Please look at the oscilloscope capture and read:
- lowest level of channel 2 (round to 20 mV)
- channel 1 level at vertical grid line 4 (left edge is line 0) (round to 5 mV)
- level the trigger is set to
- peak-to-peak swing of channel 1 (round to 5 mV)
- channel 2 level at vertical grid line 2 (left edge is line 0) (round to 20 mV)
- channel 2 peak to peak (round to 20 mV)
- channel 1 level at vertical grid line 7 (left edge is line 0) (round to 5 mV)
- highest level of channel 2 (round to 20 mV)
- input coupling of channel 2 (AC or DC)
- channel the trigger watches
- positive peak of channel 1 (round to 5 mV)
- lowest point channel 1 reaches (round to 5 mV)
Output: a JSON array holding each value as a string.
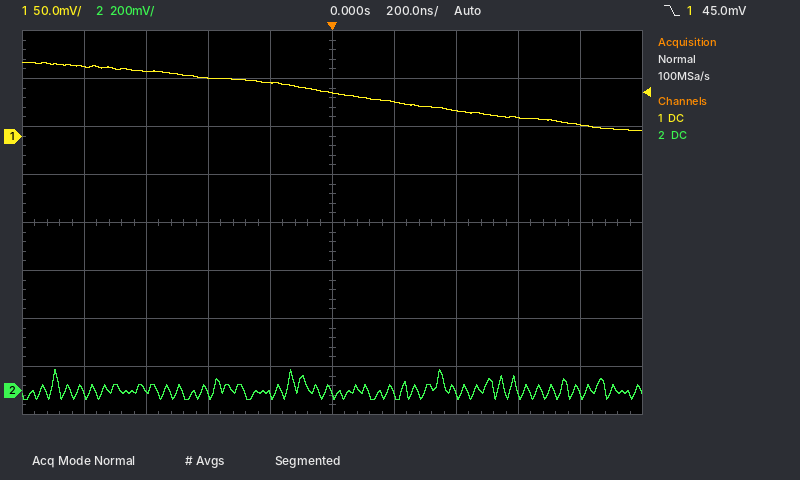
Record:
["-40 mV", "55 mV", "45.0 mV", "70 mV", "0 mV", "120 mV", "25 mV", "80 mV", "DC", "channel 1", "75 mV", "5 mV"]
